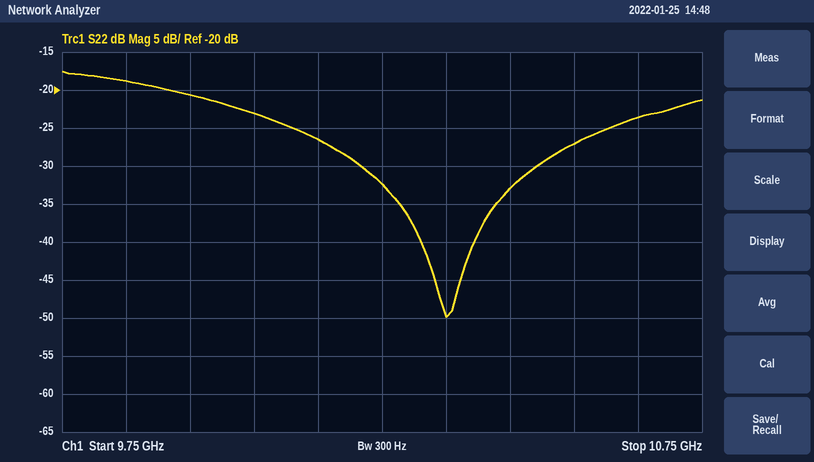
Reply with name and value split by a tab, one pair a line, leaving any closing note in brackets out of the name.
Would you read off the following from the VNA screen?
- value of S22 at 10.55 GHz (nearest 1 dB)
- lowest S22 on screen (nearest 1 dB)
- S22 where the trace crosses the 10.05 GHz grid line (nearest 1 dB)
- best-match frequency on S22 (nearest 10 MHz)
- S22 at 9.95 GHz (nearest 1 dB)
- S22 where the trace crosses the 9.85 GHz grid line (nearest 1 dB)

value of S22 at 10.55 GHz	-27 dB
lowest S22 on screen	-50 dB
S22 where the trace crosses the 10.05 GHz grid line	-23 dB
best-match frequency on S22	10.35 GHz
S22 at 9.95 GHz	-21 dB
S22 where the trace crosses the 9.85 GHz grid line	-19 dB
